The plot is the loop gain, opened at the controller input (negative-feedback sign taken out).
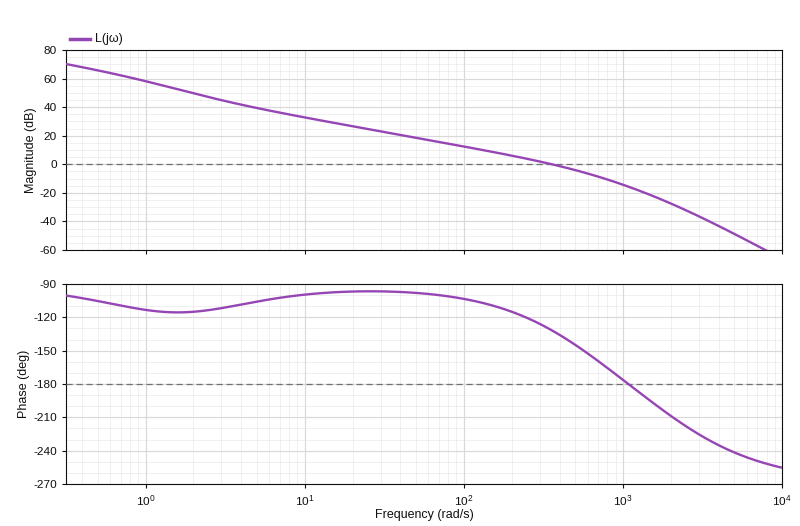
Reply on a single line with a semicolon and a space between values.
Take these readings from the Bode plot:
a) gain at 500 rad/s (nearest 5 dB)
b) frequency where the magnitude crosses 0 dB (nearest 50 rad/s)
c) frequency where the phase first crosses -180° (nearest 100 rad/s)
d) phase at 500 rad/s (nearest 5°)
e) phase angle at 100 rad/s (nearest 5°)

-5 dB; 350 rad/s; 1100 rad/s; -145°; -105°
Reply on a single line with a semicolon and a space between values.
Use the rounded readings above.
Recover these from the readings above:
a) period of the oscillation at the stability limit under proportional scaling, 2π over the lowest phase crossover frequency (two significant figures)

0.0057 s
